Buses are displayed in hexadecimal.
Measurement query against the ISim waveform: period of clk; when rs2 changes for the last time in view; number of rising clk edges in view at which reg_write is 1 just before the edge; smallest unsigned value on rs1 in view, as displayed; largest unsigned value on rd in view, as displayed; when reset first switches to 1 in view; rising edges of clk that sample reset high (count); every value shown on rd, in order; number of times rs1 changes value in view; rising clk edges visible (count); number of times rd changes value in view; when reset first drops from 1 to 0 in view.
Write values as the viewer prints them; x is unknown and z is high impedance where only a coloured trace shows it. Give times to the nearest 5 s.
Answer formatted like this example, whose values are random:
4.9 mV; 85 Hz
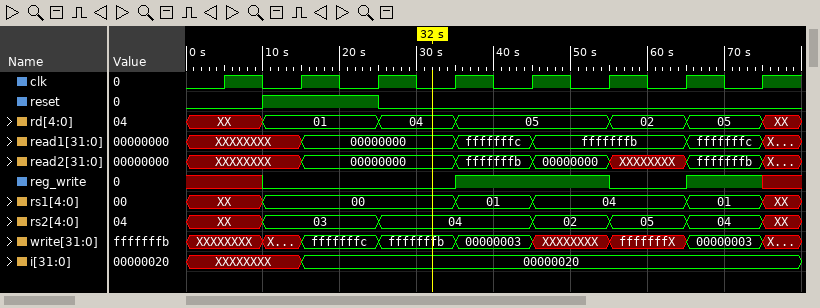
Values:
10 s; 75 s; 3; 00; 05; 10 s; 2; XX, 01, 04, 05, 02, 05, XX; 5; 8; 6; 25 s
